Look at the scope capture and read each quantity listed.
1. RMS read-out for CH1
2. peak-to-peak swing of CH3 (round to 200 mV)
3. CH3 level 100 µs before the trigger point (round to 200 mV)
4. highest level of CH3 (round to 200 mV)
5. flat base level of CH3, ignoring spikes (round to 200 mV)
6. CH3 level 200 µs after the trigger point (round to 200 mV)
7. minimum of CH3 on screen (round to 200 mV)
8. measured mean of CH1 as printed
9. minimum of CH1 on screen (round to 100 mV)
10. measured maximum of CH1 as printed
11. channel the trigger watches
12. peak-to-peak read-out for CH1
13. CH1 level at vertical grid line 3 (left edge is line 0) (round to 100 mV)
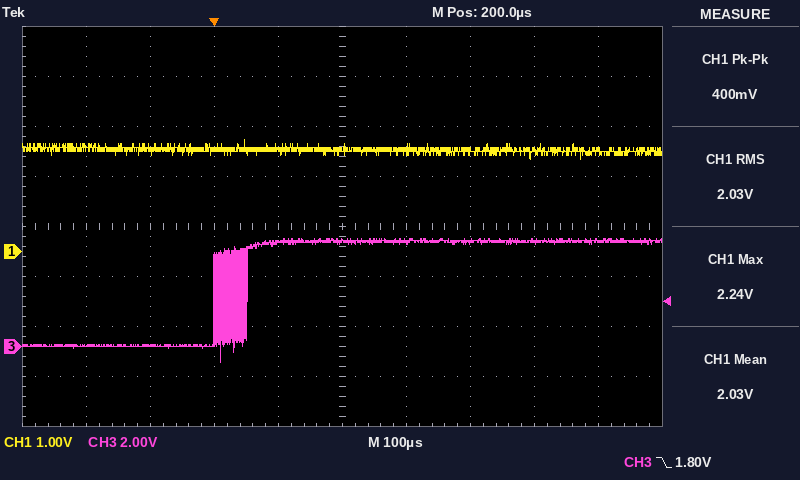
2.03 V
5.0 V
0.0 V
4.4 V
0.0 V
4.2 V
-600 mV
2.03 V
1.8 V
2.24 V
CH3
400 mV
2.0 V
